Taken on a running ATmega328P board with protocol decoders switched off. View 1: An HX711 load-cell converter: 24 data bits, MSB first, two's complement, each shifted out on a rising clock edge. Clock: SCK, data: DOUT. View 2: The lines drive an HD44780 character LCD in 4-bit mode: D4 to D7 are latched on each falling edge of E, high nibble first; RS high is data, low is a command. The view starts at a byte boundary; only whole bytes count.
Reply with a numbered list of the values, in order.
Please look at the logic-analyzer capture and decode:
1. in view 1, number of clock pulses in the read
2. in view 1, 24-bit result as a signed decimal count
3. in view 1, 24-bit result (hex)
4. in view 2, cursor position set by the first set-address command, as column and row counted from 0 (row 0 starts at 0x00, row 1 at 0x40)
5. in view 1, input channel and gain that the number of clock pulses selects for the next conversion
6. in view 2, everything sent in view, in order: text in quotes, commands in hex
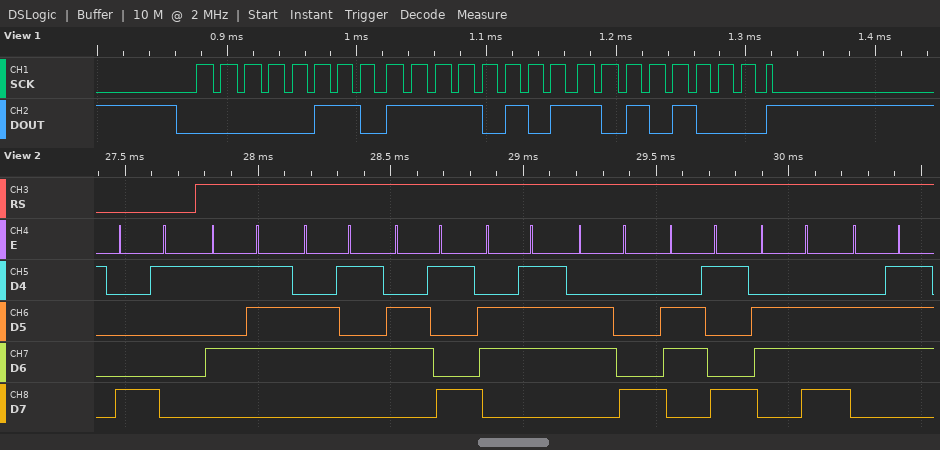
1. 25
2. 456104
3. 0x06F5A8
4. column 1, row 0
5. channel A, gain 128
6. 0x81 "Weighing"
